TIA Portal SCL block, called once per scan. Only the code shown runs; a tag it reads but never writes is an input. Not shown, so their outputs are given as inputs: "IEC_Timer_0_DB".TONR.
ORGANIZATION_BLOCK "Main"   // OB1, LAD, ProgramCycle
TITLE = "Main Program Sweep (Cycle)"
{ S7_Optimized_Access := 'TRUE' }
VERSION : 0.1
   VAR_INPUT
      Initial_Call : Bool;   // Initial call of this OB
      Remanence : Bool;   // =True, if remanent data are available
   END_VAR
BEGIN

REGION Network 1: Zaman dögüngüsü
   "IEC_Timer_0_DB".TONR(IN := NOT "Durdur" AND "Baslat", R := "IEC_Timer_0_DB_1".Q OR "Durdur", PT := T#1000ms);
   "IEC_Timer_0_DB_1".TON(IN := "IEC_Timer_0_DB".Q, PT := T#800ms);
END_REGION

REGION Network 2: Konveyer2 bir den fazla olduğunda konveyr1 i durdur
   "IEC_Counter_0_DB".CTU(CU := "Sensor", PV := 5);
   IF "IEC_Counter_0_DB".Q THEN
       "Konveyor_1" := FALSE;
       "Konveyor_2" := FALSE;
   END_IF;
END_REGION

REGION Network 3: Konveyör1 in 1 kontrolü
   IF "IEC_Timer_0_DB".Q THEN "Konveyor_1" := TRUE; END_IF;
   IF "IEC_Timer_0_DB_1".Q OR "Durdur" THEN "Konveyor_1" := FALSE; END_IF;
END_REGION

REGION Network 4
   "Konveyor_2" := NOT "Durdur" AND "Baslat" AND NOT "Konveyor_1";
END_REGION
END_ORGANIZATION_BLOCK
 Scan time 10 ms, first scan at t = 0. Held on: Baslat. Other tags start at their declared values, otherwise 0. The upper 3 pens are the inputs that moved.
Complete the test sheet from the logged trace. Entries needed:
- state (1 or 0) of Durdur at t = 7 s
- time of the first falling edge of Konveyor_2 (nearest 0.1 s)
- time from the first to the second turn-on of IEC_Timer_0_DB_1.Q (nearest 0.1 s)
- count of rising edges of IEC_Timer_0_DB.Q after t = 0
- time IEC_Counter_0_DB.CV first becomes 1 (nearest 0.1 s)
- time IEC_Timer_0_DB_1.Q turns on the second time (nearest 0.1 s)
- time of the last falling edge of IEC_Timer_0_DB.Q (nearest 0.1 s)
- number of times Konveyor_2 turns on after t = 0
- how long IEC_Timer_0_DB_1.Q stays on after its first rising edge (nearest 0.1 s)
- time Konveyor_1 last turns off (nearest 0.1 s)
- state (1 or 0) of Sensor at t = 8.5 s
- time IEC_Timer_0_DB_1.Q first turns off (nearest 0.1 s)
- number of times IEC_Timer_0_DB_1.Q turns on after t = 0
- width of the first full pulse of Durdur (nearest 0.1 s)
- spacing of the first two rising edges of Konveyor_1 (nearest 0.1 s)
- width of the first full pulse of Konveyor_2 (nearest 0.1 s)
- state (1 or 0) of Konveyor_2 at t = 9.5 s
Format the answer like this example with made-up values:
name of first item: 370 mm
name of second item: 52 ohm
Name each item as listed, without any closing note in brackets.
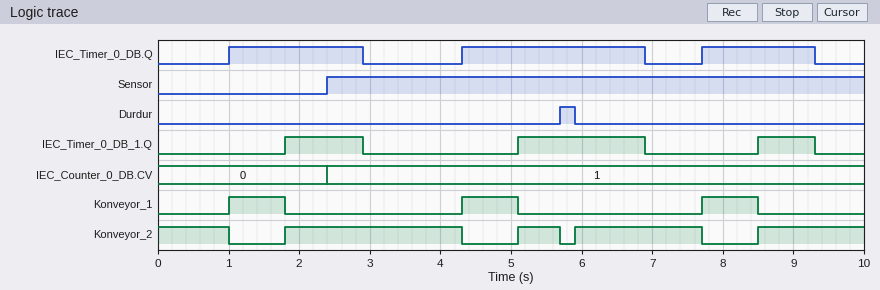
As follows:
state (1 or 0) of Durdur at t = 7 s: 0
time of the first falling edge of Konveyor_2: 1.0 s
time from the first to the second turn-on of IEC_Timer_0_DB_1.Q: 3.3 s
count of rising edges of IEC_Timer_0_DB.Q after t = 0: 3
time IEC_Counter_0_DB.CV first becomes 1: 2.4 s
time IEC_Timer_0_DB_1.Q turns on the second time: 5.1 s
time of the last falling edge of IEC_Timer_0_DB.Q: 9.3 s
number of times Konveyor_2 turns on after t = 0: 4
how long IEC_Timer_0_DB_1.Q stays on after its first rising edge: 1.1 s
time Konveyor_1 last turns off: 8.5 s
state (1 or 0) of Sensor at t = 8.5 s: 1
time IEC_Timer_0_DB_1.Q first turns off: 2.9 s
number of times IEC_Timer_0_DB_1.Q turns on after t = 0: 3
width of the first full pulse of Durdur: 0.2 s
spacing of the first two rising edges of Konveyor_1: 3.3 s
width of the first full pulse of Konveyor_2: 2.5 s
state (1 or 0) of Konveyor_2 at t = 9.5 s: 1
